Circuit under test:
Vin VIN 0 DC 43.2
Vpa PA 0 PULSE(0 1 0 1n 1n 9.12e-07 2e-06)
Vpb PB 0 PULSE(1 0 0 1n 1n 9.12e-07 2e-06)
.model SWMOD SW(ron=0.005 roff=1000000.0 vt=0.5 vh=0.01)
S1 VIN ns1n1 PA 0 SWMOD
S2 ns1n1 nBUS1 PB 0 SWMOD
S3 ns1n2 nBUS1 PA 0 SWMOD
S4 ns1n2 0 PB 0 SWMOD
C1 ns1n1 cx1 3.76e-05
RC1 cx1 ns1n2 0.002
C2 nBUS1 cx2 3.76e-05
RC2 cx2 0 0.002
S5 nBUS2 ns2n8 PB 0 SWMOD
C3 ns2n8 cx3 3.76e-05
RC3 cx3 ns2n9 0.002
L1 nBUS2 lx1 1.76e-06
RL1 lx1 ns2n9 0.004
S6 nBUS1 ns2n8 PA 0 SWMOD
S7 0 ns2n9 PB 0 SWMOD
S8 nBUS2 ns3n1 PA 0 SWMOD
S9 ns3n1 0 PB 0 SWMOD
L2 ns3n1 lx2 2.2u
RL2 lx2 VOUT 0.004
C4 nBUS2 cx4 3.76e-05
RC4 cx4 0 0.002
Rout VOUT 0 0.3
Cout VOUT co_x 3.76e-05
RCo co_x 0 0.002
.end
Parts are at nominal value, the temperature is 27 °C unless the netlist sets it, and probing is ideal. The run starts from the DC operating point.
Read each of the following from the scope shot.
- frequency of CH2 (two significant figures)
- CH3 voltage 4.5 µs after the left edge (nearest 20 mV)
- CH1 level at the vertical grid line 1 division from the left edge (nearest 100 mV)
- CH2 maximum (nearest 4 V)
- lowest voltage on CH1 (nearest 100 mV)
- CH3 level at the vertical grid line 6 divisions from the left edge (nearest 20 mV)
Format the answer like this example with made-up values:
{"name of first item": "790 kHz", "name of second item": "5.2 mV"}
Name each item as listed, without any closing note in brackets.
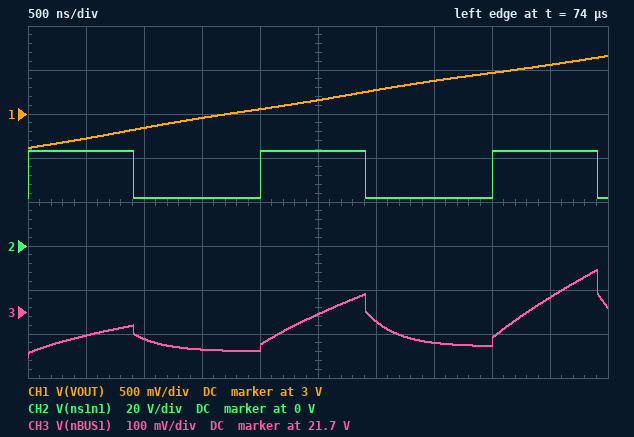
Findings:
{"frequency of CH2": "500 kHz", "CH3 voltage 4.5 µs after the left edge": "21.74 V", "CH1 level at the vertical grid line 1 division from the left edge": "2.7 V", "CH2 maximum": "44 V", "lowest voltage on CH1": "2.6 V", "CH3 level at the vertical grid line 6 divisions from the left edge": "21.68 V"}
